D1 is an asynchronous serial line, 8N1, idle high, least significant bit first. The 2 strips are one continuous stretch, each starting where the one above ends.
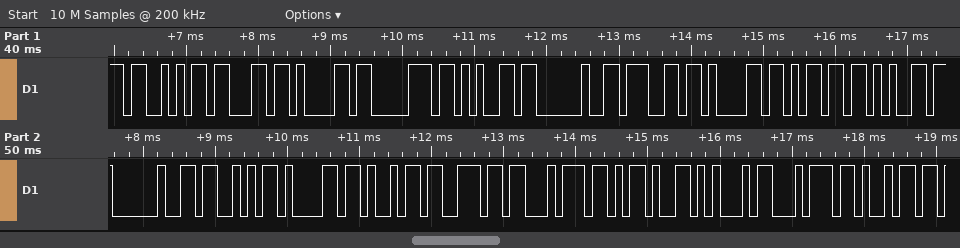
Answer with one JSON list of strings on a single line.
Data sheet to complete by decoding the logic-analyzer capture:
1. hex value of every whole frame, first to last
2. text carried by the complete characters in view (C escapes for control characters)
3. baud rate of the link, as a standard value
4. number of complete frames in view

["53 63 61 70 65 20 67 61 6D 65 20 53 61 69 6E 74 2D 45 74 69", "\"Scape game Saint-Eti\"", "9600 baud", "20"]
